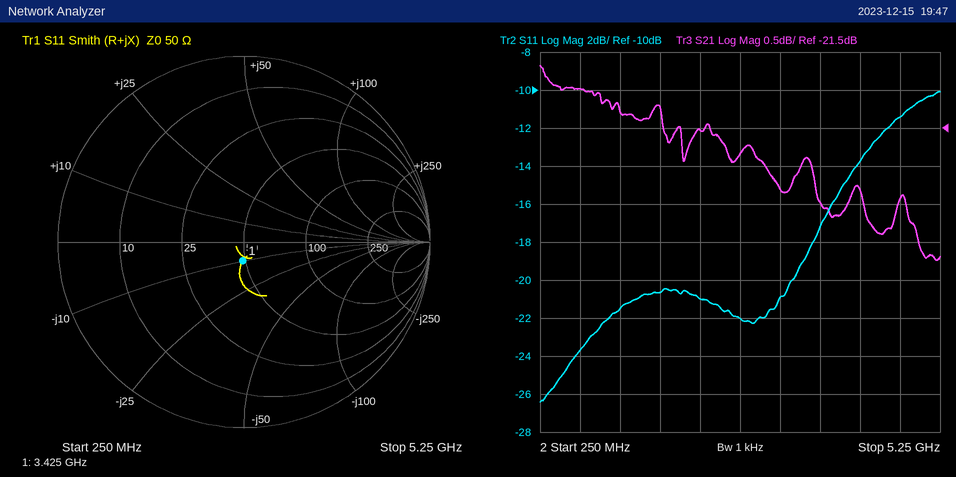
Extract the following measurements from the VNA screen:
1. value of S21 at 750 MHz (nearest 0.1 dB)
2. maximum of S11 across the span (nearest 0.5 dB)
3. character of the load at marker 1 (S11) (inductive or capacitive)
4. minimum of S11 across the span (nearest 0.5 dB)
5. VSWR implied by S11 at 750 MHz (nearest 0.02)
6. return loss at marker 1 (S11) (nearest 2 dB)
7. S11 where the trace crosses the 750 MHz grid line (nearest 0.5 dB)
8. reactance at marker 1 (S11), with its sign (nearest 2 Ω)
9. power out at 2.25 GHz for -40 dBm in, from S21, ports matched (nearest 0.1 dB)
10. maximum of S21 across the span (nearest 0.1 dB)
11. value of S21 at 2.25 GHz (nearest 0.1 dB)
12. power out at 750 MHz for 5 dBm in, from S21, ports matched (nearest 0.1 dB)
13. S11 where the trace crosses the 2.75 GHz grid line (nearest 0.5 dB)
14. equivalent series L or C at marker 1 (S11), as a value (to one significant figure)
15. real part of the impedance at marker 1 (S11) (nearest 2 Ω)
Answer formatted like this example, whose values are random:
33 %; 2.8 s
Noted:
-21.0 dB; -10.0 dB; capacitive; -26.5 dB; 1.14; 20 dB; -23.5 dB; -10 Ω; -61.5 dBm; -20.7 dB; -21.5 dB; -16.0 dBm; -22.0 dB; 5 pF; 48 Ω
